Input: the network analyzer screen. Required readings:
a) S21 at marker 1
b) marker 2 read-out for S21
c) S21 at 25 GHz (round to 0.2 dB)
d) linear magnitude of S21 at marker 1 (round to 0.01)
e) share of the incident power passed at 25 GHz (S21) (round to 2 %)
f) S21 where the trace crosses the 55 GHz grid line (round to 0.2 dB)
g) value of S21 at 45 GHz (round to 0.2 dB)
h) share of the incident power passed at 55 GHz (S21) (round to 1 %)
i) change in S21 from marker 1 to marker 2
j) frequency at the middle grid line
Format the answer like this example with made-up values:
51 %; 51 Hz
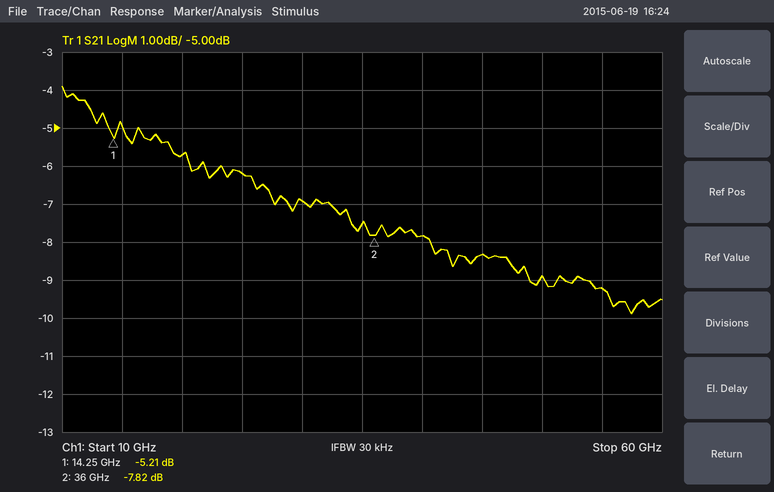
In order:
-5.21 dB; -7.82 dB; -6.2 dB; 0.55; 24 %; -9.2 dB; -8.4 dB; 12 %; -2.61 dB; 35 GHz
